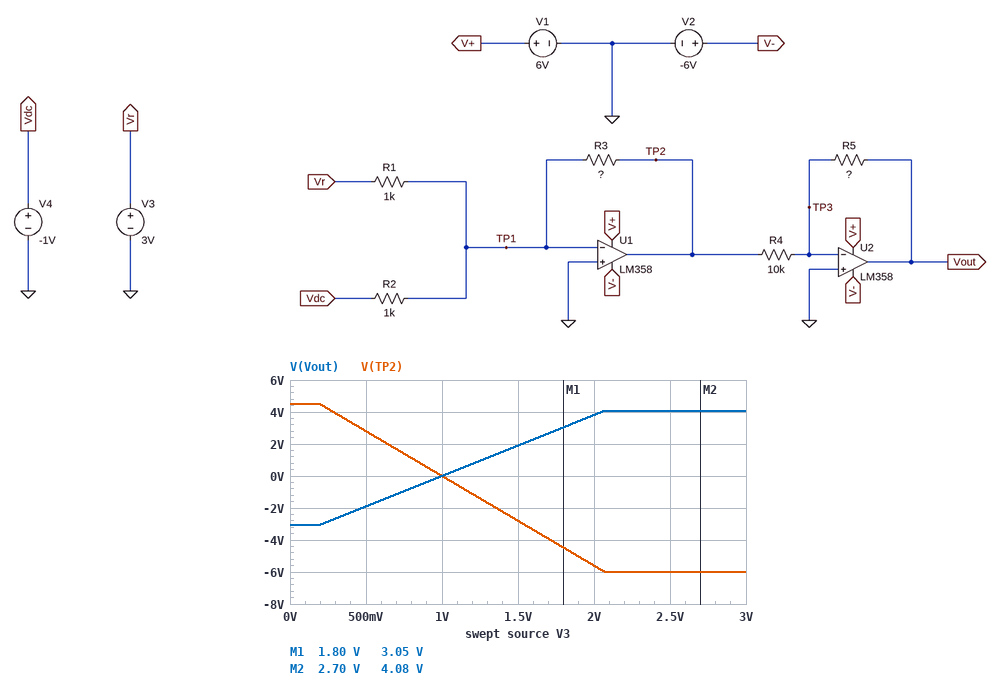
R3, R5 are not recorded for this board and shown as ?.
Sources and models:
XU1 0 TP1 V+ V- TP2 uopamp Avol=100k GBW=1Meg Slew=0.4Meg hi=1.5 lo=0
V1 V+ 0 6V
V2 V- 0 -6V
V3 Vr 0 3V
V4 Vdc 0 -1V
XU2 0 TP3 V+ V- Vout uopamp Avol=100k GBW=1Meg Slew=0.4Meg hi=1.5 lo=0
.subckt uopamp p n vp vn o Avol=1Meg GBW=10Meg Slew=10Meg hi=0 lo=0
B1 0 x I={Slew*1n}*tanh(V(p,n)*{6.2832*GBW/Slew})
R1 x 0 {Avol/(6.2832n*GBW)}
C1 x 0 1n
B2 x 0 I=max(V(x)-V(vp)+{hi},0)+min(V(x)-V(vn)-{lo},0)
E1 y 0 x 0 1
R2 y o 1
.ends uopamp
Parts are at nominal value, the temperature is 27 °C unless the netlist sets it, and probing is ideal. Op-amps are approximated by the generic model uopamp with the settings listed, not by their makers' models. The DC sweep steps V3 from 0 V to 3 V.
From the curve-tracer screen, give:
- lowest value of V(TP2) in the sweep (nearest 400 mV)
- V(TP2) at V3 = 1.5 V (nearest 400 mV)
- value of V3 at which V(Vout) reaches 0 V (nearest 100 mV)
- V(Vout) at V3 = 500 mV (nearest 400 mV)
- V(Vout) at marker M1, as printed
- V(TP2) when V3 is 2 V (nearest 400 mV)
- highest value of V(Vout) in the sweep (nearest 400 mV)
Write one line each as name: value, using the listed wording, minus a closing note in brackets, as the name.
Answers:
lowest value of V(TP2) in the sweep: -6.0 V
V(TP2) at V3 = 1.5 V: -2.8 V
value of V3 at which V(Vout) reaches 0 V: 1.0 V
V(Vout) at V3 = 500 mV: -2.0 V
V(Vout) at marker M1, as printed: 3.05 V
V(TP2) when V3 is 2 V: -5.6 V
highest value of V(Vout) in the sweep: 4.0 V
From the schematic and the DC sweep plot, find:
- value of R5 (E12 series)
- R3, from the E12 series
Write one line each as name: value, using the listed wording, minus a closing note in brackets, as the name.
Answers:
value of R5: 6.8 kΩ
R3, from the E12 series: 5.6 kΩ
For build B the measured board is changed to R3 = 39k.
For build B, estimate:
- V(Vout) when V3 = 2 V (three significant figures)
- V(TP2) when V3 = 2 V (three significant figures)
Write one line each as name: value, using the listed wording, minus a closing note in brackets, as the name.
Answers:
V(Vout) when V3 = 2 V: 4.08 V
V(TP2) when V3 = 2 V: -6.00 V
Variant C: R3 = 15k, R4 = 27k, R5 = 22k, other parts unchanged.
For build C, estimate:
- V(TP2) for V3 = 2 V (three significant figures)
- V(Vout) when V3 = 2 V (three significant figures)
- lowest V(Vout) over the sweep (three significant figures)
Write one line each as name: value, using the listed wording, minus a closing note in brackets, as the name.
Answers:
V(TP2) for V3 = 2 V: -6.00 V
V(Vout) when V3 = 2 V: 4.50 V
lowest V(Vout) over the sweep: -3.67 V
